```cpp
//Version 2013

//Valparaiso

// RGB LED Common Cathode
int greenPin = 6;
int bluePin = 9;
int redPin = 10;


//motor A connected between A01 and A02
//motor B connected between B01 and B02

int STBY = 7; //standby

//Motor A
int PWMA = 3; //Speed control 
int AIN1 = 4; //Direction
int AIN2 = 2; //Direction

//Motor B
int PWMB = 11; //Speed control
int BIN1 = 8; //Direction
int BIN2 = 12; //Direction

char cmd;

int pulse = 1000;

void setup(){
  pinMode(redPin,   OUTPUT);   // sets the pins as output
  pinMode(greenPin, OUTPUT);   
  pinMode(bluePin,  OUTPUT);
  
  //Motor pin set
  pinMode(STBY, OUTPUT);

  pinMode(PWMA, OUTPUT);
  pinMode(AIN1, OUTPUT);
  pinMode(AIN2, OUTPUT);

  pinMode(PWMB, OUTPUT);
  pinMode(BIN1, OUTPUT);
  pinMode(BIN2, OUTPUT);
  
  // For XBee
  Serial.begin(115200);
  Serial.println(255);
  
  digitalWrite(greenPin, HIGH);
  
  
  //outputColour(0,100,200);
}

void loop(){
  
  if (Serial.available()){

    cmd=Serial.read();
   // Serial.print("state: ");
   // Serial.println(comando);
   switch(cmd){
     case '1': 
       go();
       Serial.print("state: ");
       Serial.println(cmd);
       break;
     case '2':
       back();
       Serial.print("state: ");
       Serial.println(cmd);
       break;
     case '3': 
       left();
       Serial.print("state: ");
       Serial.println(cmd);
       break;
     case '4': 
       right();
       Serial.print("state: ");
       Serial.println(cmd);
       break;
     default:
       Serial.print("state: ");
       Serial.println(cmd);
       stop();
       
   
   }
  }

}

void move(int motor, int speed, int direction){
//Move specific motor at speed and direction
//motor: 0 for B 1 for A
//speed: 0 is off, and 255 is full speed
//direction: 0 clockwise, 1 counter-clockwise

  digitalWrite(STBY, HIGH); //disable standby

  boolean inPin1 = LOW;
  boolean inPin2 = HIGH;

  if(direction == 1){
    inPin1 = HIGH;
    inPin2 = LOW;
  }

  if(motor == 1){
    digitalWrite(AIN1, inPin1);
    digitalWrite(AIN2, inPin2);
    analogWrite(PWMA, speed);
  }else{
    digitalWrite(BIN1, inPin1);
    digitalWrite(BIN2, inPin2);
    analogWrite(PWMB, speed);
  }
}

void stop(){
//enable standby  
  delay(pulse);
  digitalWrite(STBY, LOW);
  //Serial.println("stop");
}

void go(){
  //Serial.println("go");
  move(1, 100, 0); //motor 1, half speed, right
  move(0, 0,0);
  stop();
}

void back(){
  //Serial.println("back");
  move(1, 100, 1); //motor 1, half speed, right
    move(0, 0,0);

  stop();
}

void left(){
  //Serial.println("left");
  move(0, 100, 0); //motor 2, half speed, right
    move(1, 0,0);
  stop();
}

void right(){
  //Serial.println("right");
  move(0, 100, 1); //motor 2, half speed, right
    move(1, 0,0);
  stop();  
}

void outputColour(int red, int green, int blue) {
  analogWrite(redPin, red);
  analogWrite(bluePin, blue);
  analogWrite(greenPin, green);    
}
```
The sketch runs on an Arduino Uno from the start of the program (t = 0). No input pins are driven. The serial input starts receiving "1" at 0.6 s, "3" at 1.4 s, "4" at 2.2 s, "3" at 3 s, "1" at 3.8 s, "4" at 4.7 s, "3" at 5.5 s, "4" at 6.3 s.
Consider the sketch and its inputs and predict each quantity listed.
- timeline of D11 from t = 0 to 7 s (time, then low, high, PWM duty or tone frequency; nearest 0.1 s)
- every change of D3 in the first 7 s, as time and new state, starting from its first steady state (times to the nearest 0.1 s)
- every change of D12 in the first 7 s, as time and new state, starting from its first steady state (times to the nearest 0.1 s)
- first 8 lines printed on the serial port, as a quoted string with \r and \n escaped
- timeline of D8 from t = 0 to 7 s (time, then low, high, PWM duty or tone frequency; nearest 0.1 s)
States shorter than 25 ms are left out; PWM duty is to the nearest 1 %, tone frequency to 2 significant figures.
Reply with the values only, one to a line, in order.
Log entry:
0 s low; 1.6 s PWM 39 %; 4.6 s low; 5.6 s PWM 39 %
0 s low; 0.6 s PWM 39 %; 1.6 s low; 4.6 s PWM 39 %; 5.6 s low
0 s low; 0.6 s high; 2.6 s low; 3.6 s high; 5.6 s low; 6.6 s high
"255\r\nstate: 1\r\nstate: 3\r\nstate: 4\r\nstate: 3\r\nstate: 1\r\nstate: 4\r\nstate: 3\r\n"
0 s low; 2.6 s high; 3.6 s low; 5.6 s high; 6.6 s low
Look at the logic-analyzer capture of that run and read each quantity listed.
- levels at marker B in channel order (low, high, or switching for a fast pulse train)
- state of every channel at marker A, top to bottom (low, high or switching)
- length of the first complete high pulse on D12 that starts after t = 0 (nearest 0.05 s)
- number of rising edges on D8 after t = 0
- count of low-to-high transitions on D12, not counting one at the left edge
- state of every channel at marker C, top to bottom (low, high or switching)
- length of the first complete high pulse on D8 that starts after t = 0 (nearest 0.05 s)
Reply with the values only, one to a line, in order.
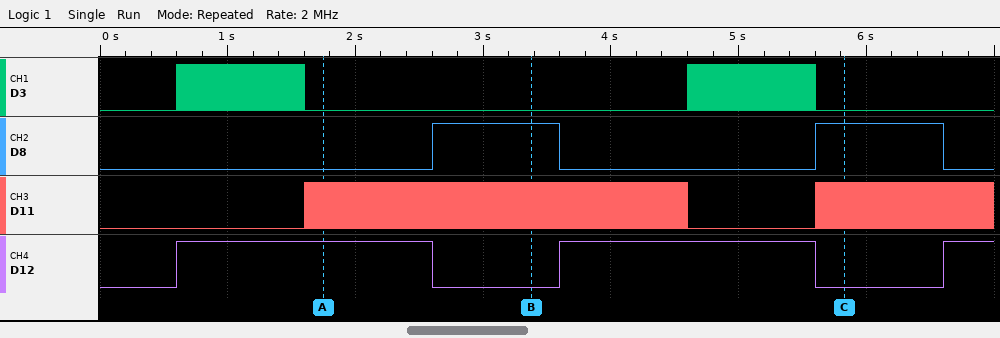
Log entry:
D3 low, D8 high, D11 switching, D12 low
D3 low, D8 low, D11 switching, D12 high
2.00 s
2
3
D3 low, D8 high, D11 switching, D12 low
1.00 s
